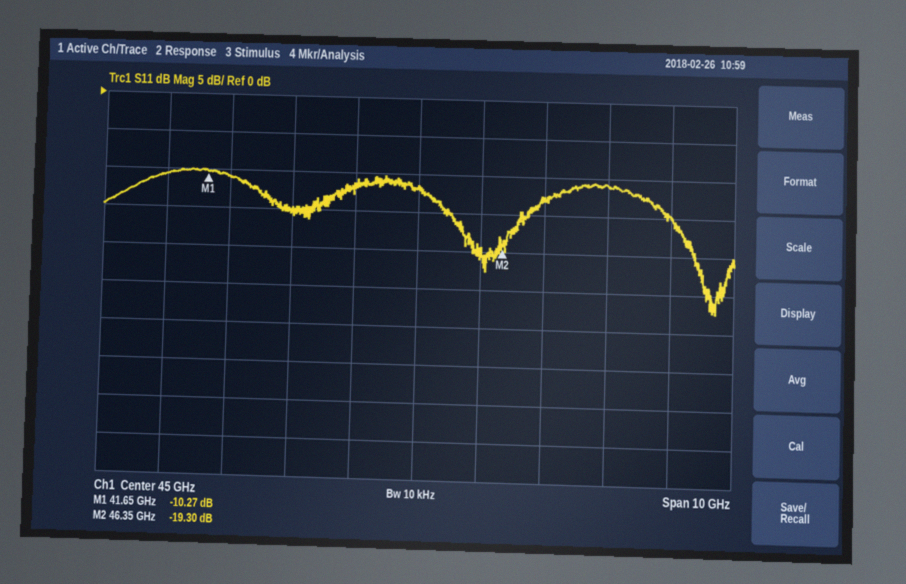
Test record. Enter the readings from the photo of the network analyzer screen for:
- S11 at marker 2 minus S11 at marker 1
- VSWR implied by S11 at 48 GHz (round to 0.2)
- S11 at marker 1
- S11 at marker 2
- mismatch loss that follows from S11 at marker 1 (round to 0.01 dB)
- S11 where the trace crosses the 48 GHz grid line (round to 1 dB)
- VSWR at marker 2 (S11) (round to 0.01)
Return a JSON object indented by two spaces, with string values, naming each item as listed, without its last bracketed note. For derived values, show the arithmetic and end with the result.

{
  "S11 at marker 2 minus S11 at marker 1": "-19.3 − (-10.27) = -9.03 dB",
  "VSWR implied by S11 at 48 GHz": "|Γ| = 10^(-11/20) = 0.2818; VSWR = (1 + 0.2818)/(1 − 0.2818) ≈ 1.8",
  "S11 at marker 1": "-10.27 dB",
  "S11 at marker 2": "-19.30 dB",
  "mismatch loss that follows from S11 at marker 1": "−10 log10(1 − 10^(-10.27/10)) ≈ 0.43 dB",
  "S11 where the trace crosses the 48 GHz grid line": "-11 dB",
  "VSWR at marker 2 (S11)": "(1 + 0.1084)/(1 − 0.1084) ≈ 1.24"
}
